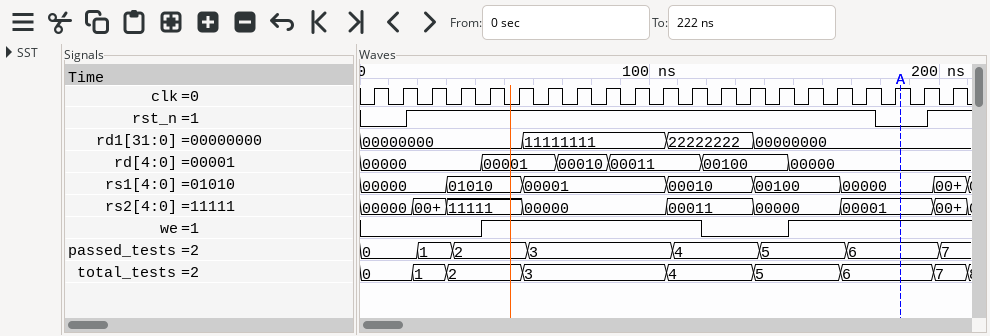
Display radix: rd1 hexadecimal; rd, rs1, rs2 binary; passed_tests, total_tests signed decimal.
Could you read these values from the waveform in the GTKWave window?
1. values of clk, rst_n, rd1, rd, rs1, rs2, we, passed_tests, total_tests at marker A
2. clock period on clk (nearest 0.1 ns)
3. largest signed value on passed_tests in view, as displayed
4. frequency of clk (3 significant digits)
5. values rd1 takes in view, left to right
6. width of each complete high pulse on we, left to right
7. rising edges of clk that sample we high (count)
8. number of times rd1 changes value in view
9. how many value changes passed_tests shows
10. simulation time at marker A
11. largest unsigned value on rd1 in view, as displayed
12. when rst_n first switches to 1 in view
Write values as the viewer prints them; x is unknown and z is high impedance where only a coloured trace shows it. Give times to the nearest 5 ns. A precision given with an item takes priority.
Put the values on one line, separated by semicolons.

clk=1, rst_n=0, rd1=00000000, rd=00000, rs1=00000, rs2=00001, we=1, passed_tests=6, total_tests=6; 10 ns; 7; 100 MHz; 00000000, 11111111, 22222222, 00000000; 75 ns; 14; 3; 7; 185 ns; 22222222; 15 ns
